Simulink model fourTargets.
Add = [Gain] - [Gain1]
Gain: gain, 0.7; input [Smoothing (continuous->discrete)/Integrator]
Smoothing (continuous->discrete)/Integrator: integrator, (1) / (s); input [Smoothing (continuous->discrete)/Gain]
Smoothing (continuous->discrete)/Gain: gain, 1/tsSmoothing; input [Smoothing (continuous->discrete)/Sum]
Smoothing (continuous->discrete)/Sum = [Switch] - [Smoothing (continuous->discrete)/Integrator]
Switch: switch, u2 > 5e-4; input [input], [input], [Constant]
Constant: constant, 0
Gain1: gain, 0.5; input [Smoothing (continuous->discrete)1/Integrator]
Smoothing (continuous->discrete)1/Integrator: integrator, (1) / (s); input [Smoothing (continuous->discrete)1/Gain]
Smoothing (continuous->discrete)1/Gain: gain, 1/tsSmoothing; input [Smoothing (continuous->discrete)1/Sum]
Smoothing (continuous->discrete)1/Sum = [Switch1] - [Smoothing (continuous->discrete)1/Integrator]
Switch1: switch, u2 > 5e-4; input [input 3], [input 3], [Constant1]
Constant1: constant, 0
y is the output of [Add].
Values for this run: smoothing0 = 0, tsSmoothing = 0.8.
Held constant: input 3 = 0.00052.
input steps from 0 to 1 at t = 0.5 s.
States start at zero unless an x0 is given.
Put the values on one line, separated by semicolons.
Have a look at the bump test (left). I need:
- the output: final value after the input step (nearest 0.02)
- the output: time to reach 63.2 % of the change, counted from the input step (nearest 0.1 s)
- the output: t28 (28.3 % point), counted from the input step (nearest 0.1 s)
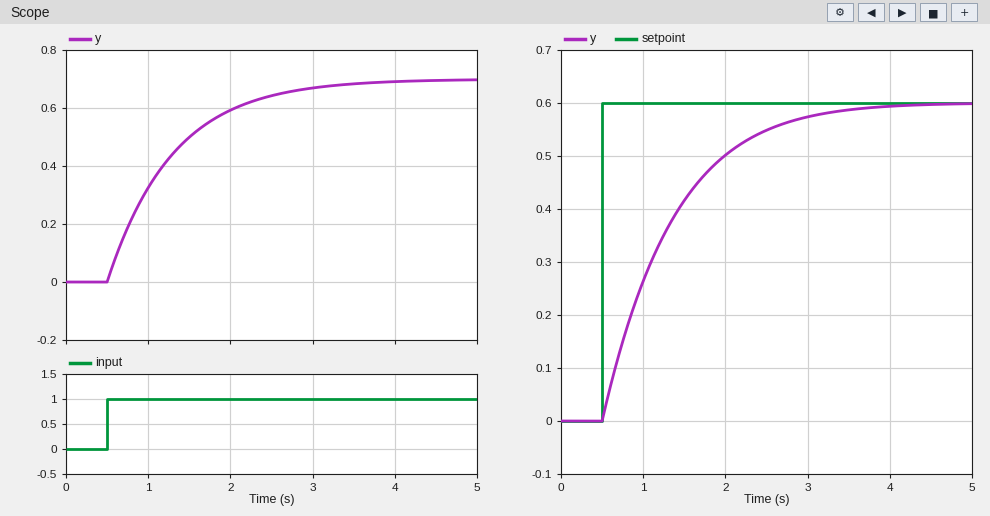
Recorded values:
0.70; 0.8 s; 0.3 s
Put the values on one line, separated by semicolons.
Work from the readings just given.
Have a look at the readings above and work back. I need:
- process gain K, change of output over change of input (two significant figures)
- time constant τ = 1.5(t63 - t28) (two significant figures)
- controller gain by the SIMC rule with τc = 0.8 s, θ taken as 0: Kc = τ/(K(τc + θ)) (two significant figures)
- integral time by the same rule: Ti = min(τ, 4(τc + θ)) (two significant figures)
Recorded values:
0.70; 0.75 s; 1.3; 0.75 s
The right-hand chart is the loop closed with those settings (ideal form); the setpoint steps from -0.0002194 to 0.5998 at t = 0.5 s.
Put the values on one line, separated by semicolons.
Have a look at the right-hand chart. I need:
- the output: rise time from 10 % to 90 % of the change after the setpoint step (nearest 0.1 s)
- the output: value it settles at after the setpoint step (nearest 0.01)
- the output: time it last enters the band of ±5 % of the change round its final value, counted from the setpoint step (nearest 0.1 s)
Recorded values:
1.8 s; 0.60; 2.4 s
